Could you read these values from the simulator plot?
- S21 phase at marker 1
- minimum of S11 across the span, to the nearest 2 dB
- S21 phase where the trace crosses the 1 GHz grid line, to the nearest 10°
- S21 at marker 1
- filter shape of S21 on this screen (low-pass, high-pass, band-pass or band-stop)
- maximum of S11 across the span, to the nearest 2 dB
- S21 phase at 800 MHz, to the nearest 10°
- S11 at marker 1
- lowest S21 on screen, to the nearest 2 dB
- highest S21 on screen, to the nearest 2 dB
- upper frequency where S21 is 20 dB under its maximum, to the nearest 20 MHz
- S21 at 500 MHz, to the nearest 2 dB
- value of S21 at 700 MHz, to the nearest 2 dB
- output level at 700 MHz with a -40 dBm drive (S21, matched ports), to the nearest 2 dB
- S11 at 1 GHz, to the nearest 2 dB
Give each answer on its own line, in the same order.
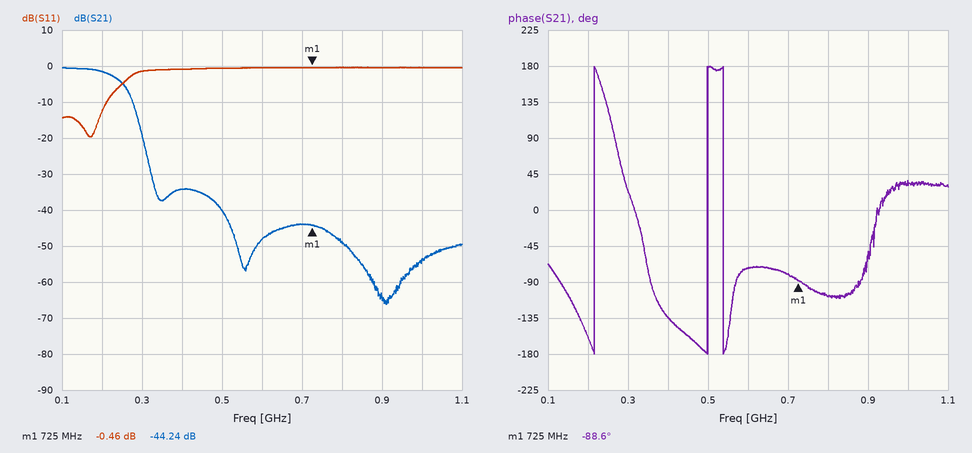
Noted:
-88.6°
-20 dB
30°
-44.24 dB
low-pass
0 dB
-110°
-0.46 dB
-66 dB
0 dB
300 MHz
-40 dB
-44 dB
-84 dBm
0 dB
